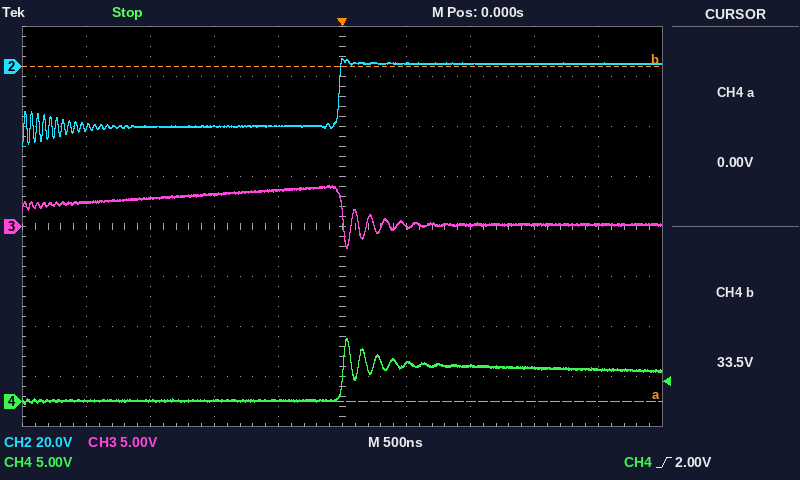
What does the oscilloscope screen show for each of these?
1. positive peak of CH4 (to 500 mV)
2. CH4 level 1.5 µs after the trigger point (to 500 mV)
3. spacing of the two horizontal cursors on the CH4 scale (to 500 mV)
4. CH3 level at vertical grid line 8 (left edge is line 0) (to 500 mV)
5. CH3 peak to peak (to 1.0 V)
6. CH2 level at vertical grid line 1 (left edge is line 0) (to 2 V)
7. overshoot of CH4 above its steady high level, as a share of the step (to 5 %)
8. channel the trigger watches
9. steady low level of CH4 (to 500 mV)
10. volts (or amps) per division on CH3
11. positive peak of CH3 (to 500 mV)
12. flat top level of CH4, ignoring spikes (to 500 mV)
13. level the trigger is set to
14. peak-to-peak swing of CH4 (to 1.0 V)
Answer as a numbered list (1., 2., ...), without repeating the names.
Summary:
1. 6.5 V
2. 3.5 V
3. 33.5 V
4. 0.0 V
5. 6.0 V
6. -24 V
7. 95 %
8. CH4
9. 0.0 V
10. 5 V
11. 4.0 V
12. 3.5 V
13. 2.00 V
14. 7.0 V
